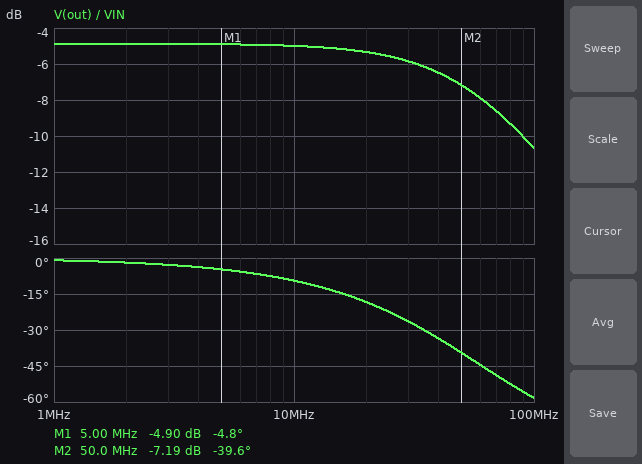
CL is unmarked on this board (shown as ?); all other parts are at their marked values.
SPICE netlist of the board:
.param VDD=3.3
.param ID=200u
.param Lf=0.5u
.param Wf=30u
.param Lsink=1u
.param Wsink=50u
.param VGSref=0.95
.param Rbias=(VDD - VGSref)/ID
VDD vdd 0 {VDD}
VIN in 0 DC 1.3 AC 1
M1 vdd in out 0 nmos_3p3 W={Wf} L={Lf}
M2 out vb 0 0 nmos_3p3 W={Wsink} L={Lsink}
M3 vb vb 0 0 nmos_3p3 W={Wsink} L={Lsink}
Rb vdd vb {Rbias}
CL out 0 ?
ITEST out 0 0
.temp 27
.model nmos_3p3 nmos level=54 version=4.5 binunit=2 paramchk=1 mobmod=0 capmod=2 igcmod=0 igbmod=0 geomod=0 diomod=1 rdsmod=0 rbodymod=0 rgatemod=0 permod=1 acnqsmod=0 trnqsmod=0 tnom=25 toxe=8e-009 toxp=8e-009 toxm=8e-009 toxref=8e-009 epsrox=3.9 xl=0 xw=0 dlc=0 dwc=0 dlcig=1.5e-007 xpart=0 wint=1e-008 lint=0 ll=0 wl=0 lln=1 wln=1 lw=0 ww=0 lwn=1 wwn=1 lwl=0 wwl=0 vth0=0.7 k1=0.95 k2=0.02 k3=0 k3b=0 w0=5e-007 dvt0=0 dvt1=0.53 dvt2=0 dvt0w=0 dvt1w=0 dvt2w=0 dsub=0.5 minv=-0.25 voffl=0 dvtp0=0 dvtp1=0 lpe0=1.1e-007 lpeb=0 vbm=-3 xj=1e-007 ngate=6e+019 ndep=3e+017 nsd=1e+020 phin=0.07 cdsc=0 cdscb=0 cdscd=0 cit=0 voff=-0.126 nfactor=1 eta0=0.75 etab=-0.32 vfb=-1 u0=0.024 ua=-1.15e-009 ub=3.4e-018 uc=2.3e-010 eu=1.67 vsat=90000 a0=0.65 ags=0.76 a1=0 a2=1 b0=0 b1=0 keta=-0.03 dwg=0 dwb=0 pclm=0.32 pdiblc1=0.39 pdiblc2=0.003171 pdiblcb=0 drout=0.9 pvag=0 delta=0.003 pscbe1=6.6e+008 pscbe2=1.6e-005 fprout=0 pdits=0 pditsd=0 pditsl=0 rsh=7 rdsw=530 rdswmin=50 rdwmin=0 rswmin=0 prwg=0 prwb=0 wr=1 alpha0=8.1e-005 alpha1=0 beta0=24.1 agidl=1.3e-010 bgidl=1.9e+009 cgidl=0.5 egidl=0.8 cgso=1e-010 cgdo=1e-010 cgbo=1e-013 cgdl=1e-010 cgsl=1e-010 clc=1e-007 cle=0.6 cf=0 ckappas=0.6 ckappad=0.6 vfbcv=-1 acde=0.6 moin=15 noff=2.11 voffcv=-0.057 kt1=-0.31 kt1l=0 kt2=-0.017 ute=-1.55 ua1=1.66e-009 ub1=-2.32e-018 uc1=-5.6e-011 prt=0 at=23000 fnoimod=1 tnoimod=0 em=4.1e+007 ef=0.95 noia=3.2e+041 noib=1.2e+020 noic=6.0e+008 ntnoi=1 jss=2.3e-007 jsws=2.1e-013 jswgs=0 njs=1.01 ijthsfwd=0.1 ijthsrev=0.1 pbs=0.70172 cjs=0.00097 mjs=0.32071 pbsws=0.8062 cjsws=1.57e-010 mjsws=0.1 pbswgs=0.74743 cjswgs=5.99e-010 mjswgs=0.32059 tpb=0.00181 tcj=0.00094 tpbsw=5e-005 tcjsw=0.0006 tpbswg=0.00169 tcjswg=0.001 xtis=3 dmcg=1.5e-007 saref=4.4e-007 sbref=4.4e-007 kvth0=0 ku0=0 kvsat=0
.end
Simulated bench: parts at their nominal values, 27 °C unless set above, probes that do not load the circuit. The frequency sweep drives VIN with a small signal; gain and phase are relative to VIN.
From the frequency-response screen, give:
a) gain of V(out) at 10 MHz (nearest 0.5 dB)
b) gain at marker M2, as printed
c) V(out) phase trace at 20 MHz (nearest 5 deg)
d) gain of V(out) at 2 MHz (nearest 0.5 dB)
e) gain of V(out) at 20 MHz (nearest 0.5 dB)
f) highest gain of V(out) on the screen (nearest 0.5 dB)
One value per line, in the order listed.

-5.0 dB
-7.19 dB
-20 deg
-5.0 dB
-5.5 dB
-5.0 dB
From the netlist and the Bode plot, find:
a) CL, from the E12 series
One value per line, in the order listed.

5.6 pF
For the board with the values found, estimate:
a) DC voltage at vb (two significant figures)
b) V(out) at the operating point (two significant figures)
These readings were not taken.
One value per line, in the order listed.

1.0 V
190 mV
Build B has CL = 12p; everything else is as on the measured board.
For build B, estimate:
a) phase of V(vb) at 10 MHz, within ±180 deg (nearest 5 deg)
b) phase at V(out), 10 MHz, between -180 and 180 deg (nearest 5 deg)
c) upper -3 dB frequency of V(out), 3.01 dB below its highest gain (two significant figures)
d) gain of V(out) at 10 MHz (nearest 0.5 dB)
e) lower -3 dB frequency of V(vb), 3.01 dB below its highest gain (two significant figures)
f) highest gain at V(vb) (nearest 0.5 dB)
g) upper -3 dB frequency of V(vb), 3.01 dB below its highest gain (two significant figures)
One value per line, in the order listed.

70 deg
-20 deg
28 MHz
-5.5 dB
26 MHz
-53.0 dB
680 MHz
